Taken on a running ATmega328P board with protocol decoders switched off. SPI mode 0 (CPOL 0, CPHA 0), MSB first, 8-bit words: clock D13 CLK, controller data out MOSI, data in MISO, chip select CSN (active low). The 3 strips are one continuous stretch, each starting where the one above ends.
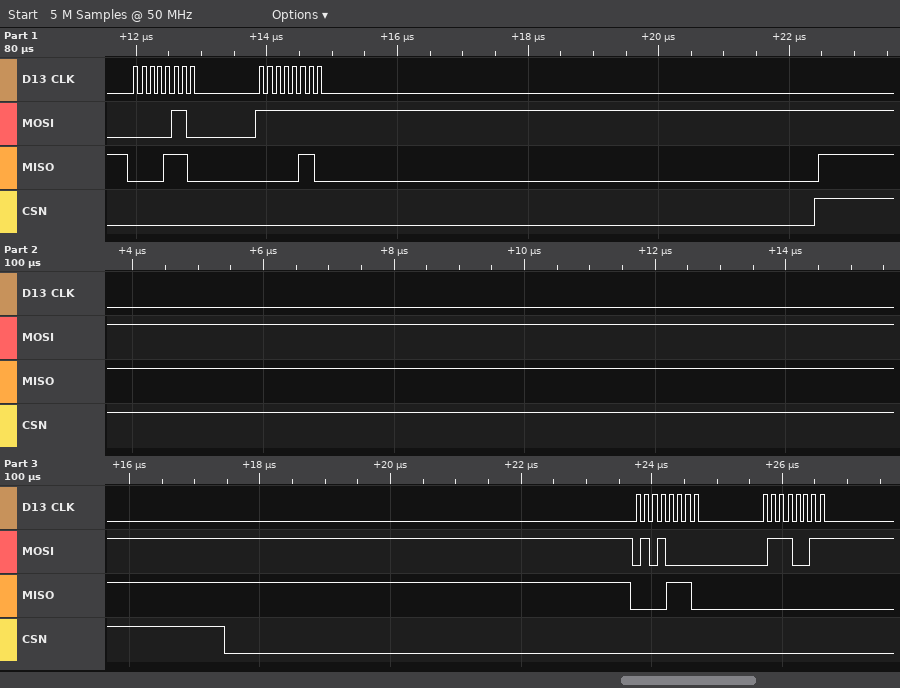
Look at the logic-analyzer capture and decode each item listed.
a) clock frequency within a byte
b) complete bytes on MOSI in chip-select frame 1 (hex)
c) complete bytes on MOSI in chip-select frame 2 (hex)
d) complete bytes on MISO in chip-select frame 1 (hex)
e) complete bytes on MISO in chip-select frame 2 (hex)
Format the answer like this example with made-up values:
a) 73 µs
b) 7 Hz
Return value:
a) 8 MHz
b) 0x06 0xFF
c) 0x50 0x73
d) 0x0E 0x06
e) 0x0E 0x00
